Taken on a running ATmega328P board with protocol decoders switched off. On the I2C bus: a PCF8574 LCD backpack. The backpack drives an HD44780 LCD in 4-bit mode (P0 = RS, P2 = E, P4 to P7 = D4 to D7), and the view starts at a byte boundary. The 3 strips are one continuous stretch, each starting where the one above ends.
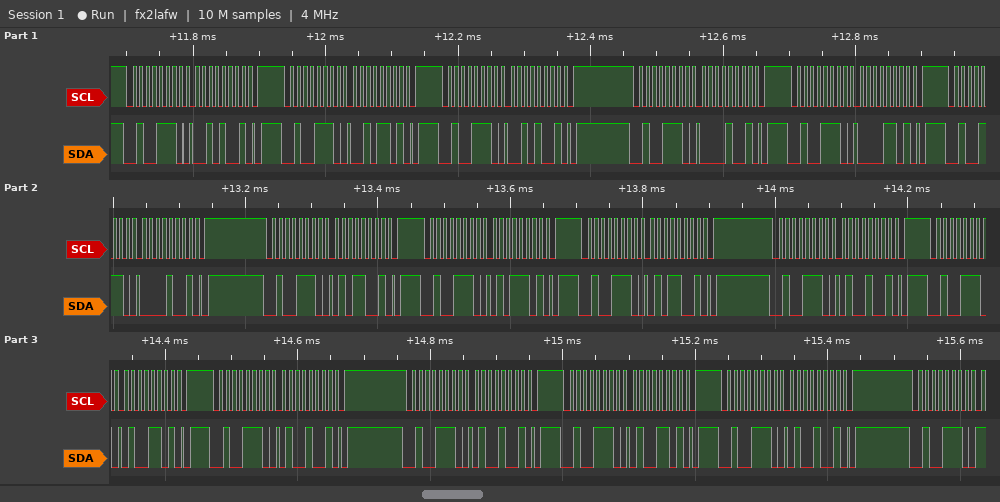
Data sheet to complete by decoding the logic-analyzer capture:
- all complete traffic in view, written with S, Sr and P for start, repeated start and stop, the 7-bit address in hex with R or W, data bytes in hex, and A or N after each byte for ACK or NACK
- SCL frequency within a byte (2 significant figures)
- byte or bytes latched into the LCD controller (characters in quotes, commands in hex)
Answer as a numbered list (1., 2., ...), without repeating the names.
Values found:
1. S 27W A 29 A P S 27W A 2D A P S 27W A 29 A P S 27W A 09 A P S 27W A 0D A P S 27W A 09 A P S 27W A 59 A P S 27W A 5D A P S 27W A 59 A P S 27W A 49 A P S 27W A 4D A P S 27W A 49 A P S 27W A 49 A P S 27W A 4D A P S 27W A 49 A P S 27W A
2. 100 kHz
3. ' ' 'T'
